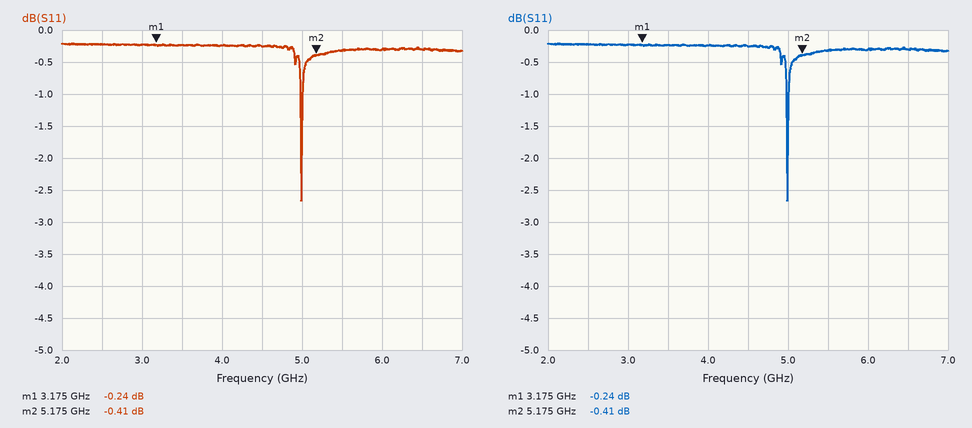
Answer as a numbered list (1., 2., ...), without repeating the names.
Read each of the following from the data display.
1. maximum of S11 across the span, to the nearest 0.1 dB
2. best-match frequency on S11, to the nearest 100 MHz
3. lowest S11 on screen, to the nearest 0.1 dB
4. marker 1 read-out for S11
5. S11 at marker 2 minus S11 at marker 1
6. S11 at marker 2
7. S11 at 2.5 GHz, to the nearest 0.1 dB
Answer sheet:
1. -0.2 dB
2. 5.0 GHz
3. -2.7 dB
4. -0.24 dB
5. -0.17 dB
6. -0.41 dB
7. -0.2 dB
